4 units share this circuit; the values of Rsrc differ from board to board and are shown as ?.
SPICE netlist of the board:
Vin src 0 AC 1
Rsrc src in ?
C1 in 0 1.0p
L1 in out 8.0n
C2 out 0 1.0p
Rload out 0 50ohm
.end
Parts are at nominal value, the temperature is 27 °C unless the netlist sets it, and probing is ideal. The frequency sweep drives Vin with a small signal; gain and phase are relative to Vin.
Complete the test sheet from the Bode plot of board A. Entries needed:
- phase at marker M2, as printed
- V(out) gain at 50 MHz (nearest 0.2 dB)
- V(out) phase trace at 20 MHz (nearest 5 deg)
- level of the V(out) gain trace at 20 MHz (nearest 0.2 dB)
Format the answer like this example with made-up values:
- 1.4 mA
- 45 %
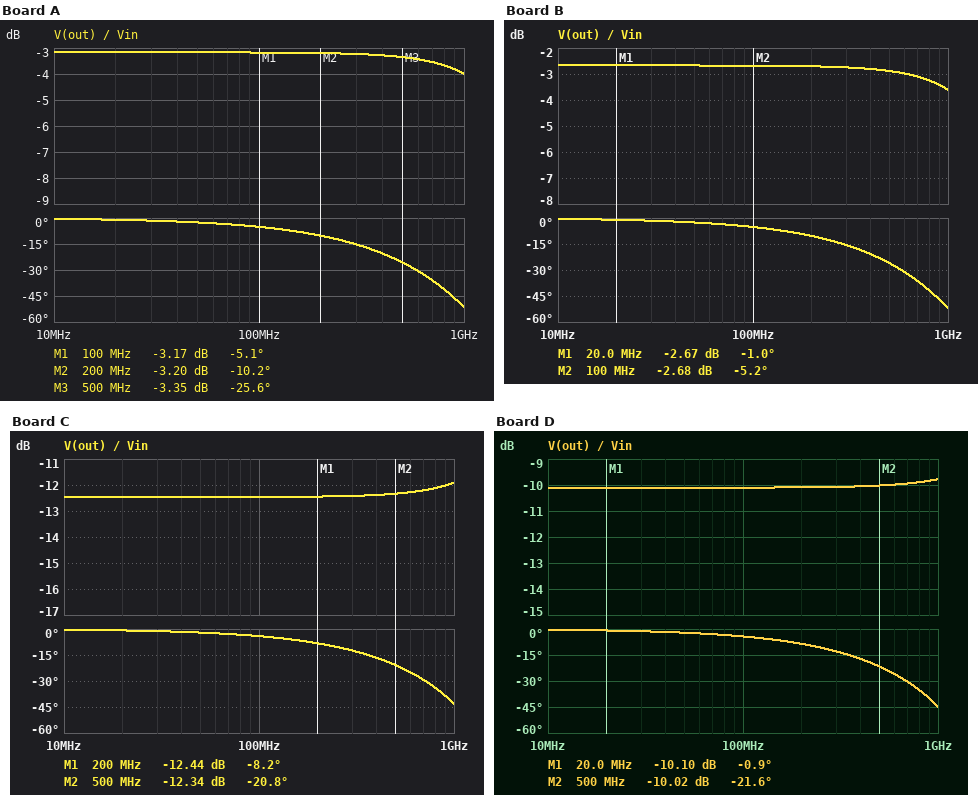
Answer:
- -10.2 deg
- -3.2 dB
- 0 deg
- -3.2 dB
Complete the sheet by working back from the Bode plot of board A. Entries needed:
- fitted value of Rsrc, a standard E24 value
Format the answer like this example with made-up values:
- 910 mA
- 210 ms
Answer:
- 22 Ω
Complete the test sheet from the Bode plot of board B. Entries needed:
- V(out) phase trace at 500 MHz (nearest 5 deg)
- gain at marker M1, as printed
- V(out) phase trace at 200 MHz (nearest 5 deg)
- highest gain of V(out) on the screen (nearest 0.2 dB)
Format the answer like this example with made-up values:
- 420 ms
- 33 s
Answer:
- -25 deg
- -2.67 dB
- -10 deg
- -2.6 dB
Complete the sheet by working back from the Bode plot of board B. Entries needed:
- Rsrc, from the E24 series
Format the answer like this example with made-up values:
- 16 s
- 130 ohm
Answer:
- 18 Ω
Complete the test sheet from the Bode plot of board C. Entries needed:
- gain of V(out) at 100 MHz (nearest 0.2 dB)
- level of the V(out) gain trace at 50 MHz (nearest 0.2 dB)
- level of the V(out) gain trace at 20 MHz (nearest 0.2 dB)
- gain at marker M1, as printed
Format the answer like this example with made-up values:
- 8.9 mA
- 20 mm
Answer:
- -12.4 dB
- -12.4 dB
- -12.4 dB
- -12.44 dB
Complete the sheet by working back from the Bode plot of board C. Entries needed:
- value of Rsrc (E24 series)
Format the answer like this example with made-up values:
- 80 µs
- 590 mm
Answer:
- 160 Ω
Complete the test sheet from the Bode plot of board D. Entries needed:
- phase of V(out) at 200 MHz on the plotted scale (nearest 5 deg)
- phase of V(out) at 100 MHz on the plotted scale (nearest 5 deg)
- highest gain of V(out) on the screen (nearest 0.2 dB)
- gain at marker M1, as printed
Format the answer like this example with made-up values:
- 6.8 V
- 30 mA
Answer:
- -10 deg
- -5 deg
- -9.8 dB
- -10.10 dB
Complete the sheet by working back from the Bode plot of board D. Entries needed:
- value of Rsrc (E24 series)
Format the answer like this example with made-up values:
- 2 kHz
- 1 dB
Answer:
- 110 Ω
